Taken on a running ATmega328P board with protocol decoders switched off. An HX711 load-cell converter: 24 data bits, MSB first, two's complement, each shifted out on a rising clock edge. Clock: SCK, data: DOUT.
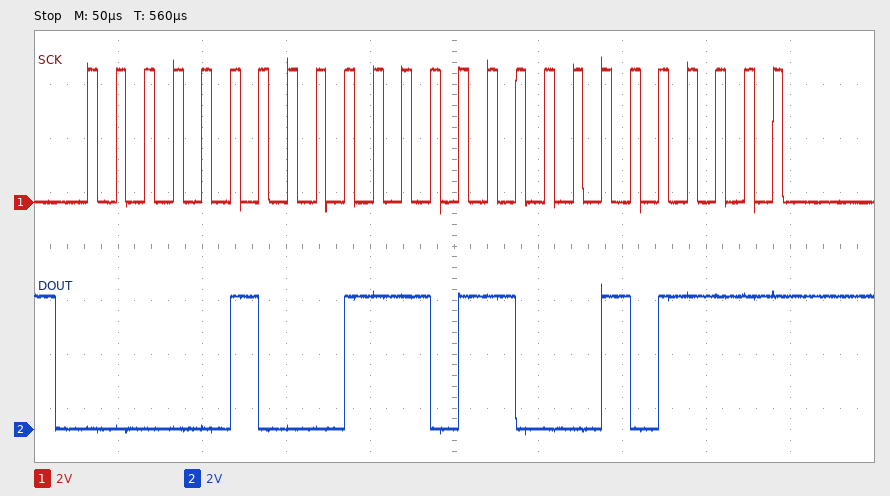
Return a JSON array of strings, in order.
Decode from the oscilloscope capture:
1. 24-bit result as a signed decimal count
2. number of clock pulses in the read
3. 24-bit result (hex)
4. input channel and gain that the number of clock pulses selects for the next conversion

["292399", "25", "0x04762F", "channel A, gain 128"]
